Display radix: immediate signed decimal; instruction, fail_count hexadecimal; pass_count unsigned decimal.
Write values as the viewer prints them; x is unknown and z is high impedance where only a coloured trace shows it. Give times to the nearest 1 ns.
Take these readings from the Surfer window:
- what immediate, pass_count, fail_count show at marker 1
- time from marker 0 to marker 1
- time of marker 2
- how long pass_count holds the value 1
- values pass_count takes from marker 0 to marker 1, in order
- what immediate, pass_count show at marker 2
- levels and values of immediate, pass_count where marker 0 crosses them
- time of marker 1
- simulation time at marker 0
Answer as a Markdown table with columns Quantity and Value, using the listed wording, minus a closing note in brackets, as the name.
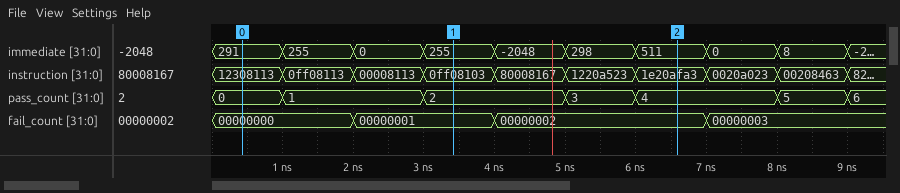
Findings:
| Quantity | Value |
|---|---|
| what immediate, pass_count, fail_count show at marker 1 | immediate=255, pass_count=2, fail_count=00000001 |
| time from marker 0 to marker 1 | 3 ns |
| time of marker 2 | 7 ns |
| how long pass_count holds the value 1 | 2 ns |
| values pass_count takes from marker 0 to marker 1, in order | 0, 1, 2 |
| what immediate, pass_count show at marker 2 | immediate=511, pass_count=4 |
| levels and values of immediate, pass_count where marker 0 crosses them | immediate=291, pass_count=0 |
| time of marker 1 | 3 ns |
| simulation time at marker 0 | 0 ns |
